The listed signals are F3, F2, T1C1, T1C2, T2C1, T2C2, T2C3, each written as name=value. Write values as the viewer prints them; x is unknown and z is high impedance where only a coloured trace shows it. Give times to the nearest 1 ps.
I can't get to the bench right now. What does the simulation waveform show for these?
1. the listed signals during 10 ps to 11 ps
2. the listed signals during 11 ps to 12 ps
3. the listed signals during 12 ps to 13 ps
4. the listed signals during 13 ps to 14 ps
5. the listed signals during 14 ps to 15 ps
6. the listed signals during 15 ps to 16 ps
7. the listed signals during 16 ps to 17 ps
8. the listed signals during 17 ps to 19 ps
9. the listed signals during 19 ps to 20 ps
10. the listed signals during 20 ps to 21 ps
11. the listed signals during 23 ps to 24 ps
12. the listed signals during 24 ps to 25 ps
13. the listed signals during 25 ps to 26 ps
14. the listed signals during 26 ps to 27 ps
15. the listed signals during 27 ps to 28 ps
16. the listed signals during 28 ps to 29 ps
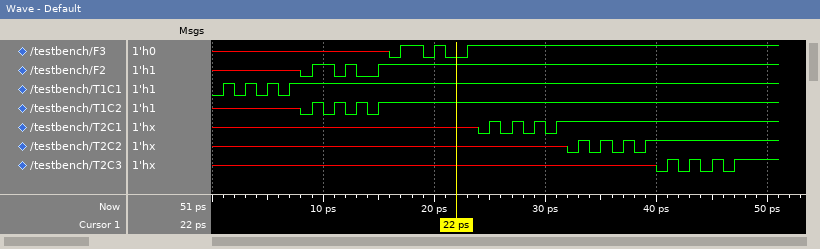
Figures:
F3=x, F2=1, T1C1=1, T1C2=0, T2C1=x, T2C2=x, T2C3=x
F3=x, F2=0, T1C1=1, T1C2=1, T2C1=x, T2C2=x, T2C3=x
F3=x, F2=1, T1C1=1, T1C2=0, T2C1=x, T2C2=x, T2C3=x
F3=x, F2=0, T1C1=1, T1C2=1, T2C1=x, T2C2=x, T2C3=x
F3=x, F2=0, T1C1=1, T1C2=0, T2C1=x, T2C2=x, T2C3=x
F3=x, F2=1, T1C1=1, T1C2=1, T2C1=x, T2C2=x, T2C3=x
F3=0, F2=1, T1C1=1, T1C2=1, T2C1=x, T2C2=x, T2C3=x
F3=1, F2=1, T1C1=1, T1C2=1, T2C1=x, T2C2=x, T2C3=x
F3=0, F2=1, T1C1=1, T1C2=1, T2C1=x, T2C2=x, T2C3=x
F3=1, F2=1, T1C1=1, T1C2=1, T2C1=x, T2C2=x, T2C3=x
F3=1, F2=1, T1C1=1, T1C2=1, T2C1=x, T2C2=x, T2C3=x
F3=1, F2=1, T1C1=1, T1C2=1, T2C1=0, T2C2=x, T2C3=x
F3=1, F2=1, T1C1=1, T1C2=1, T2C1=1, T2C2=x, T2C3=x
F3=1, F2=1, T1C1=1, T1C2=1, T2C1=0, T2C2=x, T2C3=x
F3=1, F2=1, T1C1=1, T1C2=1, T2C1=1, T2C2=x, T2C3=x
F3=1, F2=1, T1C1=1, T1C2=1, T2C1=0, T2C2=x, T2C3=x
